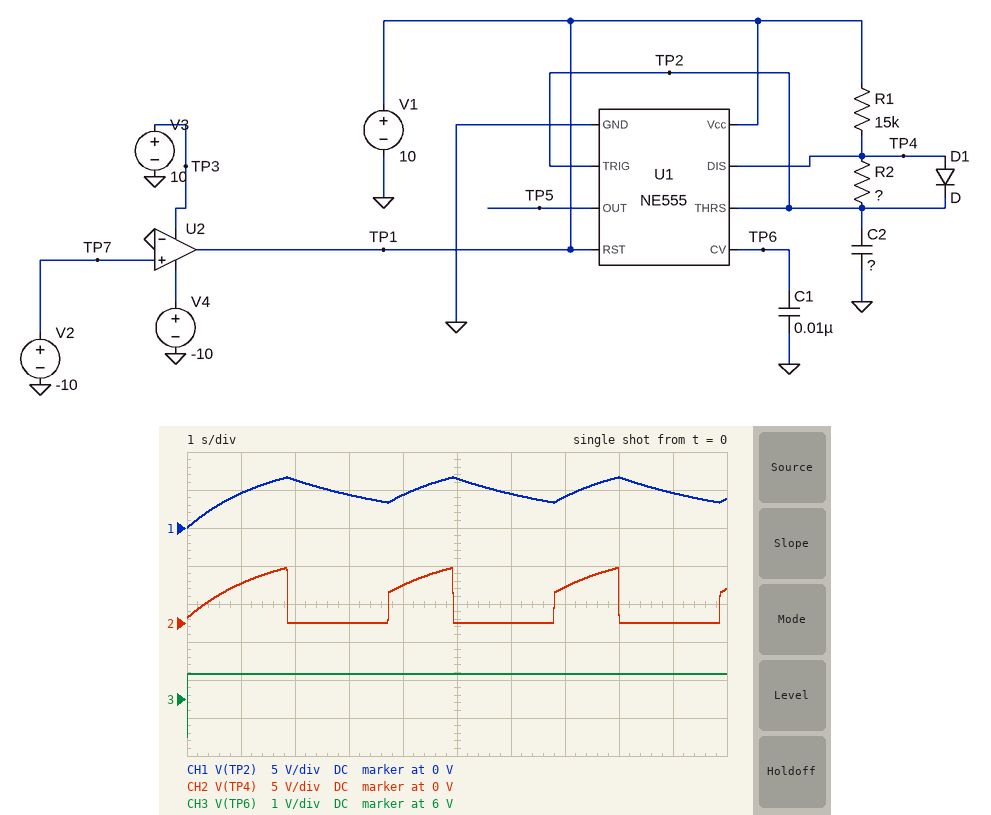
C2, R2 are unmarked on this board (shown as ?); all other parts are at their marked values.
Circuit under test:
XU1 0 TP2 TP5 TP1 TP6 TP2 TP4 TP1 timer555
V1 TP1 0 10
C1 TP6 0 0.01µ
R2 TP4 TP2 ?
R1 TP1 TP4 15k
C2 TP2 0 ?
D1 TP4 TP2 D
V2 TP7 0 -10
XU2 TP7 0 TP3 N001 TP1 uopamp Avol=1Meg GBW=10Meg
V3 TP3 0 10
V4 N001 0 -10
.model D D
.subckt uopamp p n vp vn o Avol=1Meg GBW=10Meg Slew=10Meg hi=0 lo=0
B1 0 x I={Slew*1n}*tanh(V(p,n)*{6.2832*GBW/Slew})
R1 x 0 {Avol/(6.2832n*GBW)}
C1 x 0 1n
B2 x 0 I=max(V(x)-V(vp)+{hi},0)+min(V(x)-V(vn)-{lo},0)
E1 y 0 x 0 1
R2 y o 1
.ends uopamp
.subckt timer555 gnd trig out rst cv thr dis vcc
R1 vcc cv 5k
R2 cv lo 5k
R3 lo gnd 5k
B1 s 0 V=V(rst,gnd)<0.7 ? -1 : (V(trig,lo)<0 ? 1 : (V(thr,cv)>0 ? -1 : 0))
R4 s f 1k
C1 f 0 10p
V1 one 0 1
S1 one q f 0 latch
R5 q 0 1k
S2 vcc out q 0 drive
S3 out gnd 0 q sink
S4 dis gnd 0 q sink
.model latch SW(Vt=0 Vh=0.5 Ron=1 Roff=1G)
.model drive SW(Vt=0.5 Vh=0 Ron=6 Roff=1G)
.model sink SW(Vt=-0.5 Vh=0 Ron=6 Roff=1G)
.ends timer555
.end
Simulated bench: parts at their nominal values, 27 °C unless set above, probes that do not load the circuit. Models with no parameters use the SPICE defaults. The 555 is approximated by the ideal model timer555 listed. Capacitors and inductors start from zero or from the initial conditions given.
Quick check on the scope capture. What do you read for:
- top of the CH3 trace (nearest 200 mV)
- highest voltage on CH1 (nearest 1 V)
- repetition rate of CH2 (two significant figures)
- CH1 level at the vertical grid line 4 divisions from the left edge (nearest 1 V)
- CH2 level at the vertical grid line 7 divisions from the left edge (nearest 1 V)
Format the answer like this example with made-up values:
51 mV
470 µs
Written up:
6.6 V
7 V
320 mHz
4 V
5 V
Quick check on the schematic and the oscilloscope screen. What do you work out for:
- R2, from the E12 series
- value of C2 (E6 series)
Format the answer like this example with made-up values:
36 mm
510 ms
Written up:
27 kΩ
100 µF
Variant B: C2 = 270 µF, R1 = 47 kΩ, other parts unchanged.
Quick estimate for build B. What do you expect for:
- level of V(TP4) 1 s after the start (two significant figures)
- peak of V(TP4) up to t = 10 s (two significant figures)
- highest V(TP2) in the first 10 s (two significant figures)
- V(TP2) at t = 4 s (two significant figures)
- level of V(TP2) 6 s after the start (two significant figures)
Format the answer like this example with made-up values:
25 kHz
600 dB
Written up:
1.3 V
5.7 V
5.1 V
2.5 V
3.5 V
